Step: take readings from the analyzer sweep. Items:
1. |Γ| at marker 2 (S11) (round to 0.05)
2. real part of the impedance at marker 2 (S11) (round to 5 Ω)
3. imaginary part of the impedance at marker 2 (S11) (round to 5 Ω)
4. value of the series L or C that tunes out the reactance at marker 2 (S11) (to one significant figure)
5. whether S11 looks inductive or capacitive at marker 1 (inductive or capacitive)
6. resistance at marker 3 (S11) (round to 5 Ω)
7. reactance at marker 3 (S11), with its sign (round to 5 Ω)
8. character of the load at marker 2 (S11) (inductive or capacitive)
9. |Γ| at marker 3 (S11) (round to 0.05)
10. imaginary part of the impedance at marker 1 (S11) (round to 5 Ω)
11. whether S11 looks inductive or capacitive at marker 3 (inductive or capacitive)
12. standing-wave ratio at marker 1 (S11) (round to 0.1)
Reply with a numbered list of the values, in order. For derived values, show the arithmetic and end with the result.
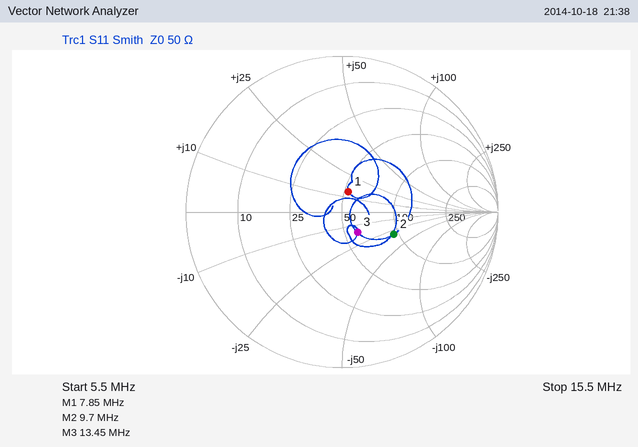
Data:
1. 0.35
2. 95 Ω
3. -30 Ω
4. L = 30 Ω/(2π × 9.7 MHz) ≈ 492 nH, so 500 nH to one significant figure
5. inductive
6. 60 Ω
7. -15 Ω
8. capacitive
9. 0.15
10. +15 Ω
11. capacitive
12. 1.3
